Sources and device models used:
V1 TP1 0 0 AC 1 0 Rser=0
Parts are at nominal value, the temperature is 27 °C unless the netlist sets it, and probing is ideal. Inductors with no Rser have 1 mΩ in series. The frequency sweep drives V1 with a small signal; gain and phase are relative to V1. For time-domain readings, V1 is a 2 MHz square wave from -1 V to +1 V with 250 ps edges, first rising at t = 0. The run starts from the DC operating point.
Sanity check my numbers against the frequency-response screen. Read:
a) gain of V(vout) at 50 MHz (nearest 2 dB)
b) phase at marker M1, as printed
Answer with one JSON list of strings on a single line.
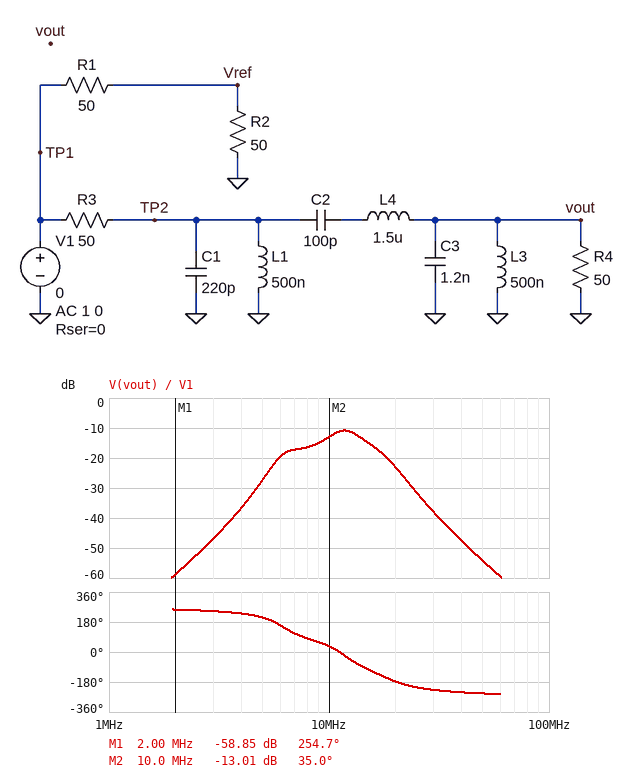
["-54 dB", "254.7 deg"]
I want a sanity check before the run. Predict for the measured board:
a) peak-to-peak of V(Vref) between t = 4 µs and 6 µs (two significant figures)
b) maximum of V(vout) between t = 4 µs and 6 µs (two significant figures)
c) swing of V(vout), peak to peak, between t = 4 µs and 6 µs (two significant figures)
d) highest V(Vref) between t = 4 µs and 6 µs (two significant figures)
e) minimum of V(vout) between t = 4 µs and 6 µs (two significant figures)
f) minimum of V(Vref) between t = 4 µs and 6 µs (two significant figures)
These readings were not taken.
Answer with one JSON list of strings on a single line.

["1.0 V", "150 mV", "300 mV", "500 mV", "-150 mV", "-500 mV"]
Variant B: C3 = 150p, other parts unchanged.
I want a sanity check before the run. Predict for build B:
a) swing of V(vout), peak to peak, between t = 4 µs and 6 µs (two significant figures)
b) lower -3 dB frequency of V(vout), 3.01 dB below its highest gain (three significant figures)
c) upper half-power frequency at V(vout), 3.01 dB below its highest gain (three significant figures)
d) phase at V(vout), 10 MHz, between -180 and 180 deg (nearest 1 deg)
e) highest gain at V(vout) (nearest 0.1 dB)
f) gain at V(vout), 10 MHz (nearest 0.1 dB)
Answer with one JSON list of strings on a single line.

["630 mV", "9.09 MHz", "20.4 MHz", "107 deg", "-6.1 dB", "-6.5 dB"]
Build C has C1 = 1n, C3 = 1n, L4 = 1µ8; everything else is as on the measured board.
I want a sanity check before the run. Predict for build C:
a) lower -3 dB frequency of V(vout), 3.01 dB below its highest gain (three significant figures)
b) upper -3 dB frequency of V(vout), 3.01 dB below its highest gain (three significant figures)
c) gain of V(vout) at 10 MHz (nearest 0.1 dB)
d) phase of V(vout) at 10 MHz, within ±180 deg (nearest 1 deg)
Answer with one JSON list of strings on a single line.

["12.8 MHz", "13.7 MHz", "-16.3 dB", "-42 deg"]
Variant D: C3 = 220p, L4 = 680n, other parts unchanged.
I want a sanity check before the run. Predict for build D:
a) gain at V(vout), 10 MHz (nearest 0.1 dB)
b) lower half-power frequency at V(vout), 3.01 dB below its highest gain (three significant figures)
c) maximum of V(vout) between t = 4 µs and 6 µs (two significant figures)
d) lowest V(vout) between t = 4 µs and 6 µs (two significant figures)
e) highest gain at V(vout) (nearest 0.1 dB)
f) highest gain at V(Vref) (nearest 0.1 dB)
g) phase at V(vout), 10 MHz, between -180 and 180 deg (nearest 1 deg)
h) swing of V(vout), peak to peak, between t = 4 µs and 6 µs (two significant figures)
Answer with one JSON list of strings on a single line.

["-9.9 dB", "10.4 MHz", "370 mV", "-370 mV", "-6.0 dB", "-6.0 dB", "134 deg", "740 mV"]
